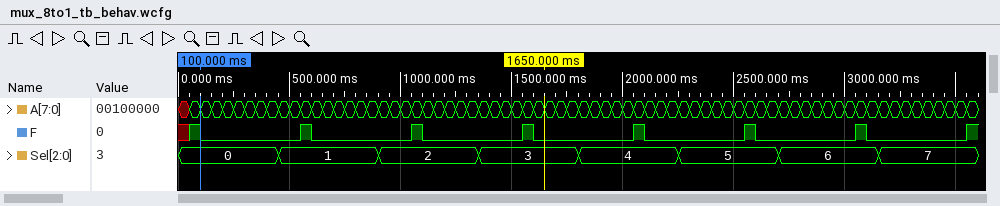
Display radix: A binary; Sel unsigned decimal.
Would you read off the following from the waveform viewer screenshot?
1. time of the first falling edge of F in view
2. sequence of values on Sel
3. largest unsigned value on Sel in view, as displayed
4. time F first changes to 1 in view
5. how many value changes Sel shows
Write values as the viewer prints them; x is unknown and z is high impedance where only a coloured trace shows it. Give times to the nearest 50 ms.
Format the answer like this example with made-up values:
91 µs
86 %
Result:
100 ms
0, 1, 2, 3, 4, 5, 6, 7
7
50 ms
7
